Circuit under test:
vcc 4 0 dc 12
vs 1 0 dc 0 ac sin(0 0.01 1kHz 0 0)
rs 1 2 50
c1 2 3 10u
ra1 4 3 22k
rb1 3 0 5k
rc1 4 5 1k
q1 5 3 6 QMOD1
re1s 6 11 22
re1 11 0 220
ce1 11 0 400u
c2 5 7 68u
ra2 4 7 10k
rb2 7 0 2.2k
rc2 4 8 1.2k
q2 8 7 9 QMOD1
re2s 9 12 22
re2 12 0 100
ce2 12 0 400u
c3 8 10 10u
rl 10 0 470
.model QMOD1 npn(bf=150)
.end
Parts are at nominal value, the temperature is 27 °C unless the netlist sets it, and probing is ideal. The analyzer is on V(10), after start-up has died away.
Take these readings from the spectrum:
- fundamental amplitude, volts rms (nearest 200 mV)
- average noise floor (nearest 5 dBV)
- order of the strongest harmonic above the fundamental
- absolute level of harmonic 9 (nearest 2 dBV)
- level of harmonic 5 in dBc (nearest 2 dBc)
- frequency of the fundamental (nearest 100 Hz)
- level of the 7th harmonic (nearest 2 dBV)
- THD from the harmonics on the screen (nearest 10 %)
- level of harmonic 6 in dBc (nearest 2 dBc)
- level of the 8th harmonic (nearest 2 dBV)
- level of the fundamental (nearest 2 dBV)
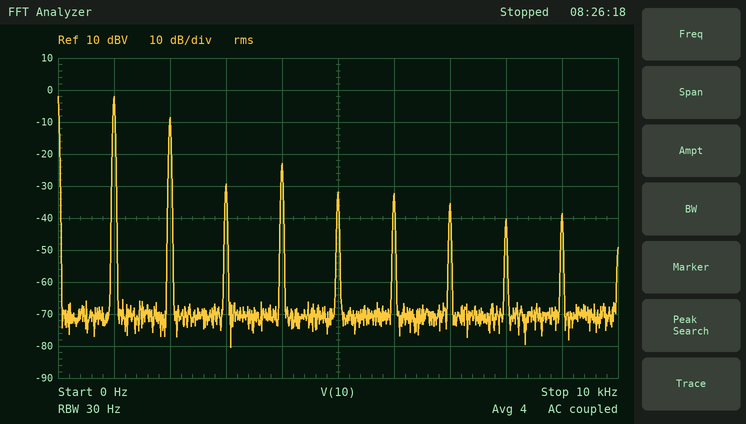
800 mV
-70 dBV
2
-38 dBV
-30 dBc
1.0 kHz
-36 dBV
50 %
-30 dBc
-40 dBV
-2 dBV
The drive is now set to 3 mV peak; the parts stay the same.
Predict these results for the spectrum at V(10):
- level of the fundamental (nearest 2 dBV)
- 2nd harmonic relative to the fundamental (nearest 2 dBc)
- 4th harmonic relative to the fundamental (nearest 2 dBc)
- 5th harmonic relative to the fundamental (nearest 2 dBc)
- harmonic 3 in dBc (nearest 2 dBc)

-20 dBV
-4 dBc
-18 dBc
-36 dBc
-10 dBc
